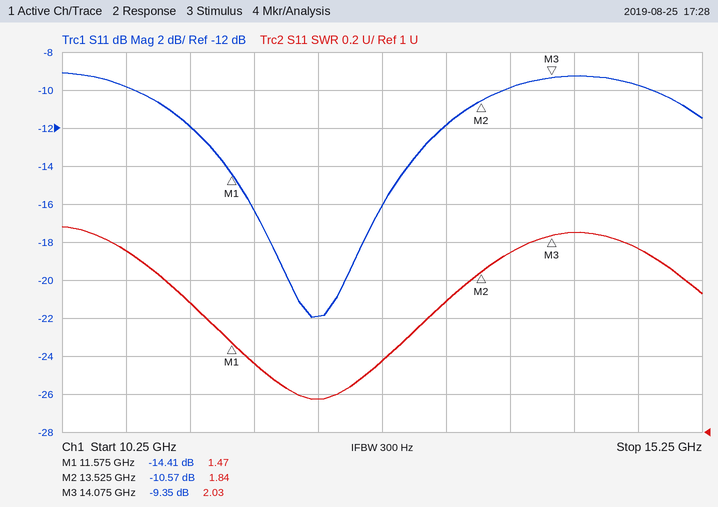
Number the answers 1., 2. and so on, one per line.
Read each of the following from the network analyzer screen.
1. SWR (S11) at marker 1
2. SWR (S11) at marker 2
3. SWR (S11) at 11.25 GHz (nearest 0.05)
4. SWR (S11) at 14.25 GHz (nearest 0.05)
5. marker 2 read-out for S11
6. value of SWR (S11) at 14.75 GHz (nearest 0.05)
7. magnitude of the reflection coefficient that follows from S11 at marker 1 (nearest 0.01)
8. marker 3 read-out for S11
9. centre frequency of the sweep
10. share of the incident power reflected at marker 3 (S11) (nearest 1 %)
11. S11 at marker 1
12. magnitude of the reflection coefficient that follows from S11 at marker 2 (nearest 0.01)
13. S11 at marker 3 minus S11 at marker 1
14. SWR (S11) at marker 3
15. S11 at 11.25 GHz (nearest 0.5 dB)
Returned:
1. 1.47
2. 1.84
3. 1.70
4. 2.05
5. -10.57 dB
6. 1.95
7. 0.19
8. -9.35 dB
9. 12.75 GHz
10. 12 %
11. -14.41 dB
12. 0.30
13. 5.06 dB
14. 2.03
15. -12.0 dB
